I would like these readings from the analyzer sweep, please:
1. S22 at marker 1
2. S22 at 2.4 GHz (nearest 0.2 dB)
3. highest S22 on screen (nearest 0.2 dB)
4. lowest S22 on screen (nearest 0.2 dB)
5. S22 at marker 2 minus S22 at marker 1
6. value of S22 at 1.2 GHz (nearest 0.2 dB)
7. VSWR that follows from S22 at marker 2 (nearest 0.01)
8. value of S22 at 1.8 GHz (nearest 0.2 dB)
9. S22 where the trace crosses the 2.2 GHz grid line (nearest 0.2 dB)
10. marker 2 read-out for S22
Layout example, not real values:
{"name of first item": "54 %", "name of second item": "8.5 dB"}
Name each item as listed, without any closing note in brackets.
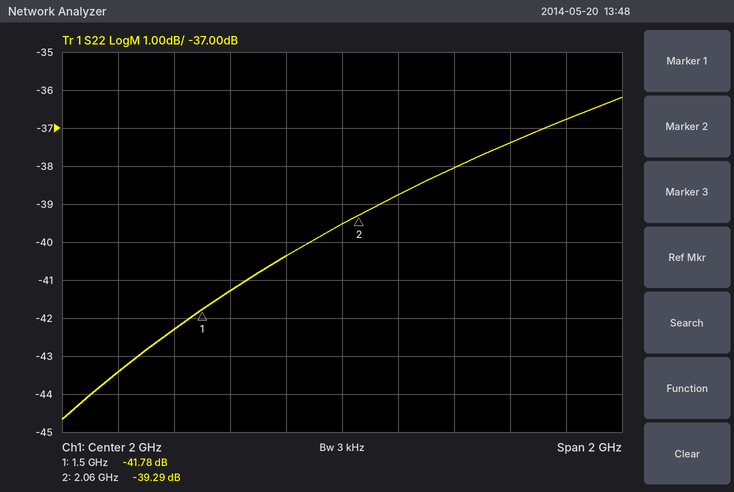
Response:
{"S22 at marker 1": "-41.78 dB", "S22 at 2.4 GHz": "-38.0 dB", "highest S22 on screen": "-36.2 dB", "lowest S22 on screen": "-44.6 dB", "S22 at marker 2 minus S22 at marker 1": "2.49 dB", "value of S22 at 1.2 GHz": "-43.4 dB", "VSWR that follows from S22 at marker 2": "1.02", "value of S22 at 1.8 GHz": "-40.4 dB", "S22 where the trace crosses the 2.2 GHz grid line": "-38.8 dB", "marker 2 read-out for S22": "-39.29 dB"}
